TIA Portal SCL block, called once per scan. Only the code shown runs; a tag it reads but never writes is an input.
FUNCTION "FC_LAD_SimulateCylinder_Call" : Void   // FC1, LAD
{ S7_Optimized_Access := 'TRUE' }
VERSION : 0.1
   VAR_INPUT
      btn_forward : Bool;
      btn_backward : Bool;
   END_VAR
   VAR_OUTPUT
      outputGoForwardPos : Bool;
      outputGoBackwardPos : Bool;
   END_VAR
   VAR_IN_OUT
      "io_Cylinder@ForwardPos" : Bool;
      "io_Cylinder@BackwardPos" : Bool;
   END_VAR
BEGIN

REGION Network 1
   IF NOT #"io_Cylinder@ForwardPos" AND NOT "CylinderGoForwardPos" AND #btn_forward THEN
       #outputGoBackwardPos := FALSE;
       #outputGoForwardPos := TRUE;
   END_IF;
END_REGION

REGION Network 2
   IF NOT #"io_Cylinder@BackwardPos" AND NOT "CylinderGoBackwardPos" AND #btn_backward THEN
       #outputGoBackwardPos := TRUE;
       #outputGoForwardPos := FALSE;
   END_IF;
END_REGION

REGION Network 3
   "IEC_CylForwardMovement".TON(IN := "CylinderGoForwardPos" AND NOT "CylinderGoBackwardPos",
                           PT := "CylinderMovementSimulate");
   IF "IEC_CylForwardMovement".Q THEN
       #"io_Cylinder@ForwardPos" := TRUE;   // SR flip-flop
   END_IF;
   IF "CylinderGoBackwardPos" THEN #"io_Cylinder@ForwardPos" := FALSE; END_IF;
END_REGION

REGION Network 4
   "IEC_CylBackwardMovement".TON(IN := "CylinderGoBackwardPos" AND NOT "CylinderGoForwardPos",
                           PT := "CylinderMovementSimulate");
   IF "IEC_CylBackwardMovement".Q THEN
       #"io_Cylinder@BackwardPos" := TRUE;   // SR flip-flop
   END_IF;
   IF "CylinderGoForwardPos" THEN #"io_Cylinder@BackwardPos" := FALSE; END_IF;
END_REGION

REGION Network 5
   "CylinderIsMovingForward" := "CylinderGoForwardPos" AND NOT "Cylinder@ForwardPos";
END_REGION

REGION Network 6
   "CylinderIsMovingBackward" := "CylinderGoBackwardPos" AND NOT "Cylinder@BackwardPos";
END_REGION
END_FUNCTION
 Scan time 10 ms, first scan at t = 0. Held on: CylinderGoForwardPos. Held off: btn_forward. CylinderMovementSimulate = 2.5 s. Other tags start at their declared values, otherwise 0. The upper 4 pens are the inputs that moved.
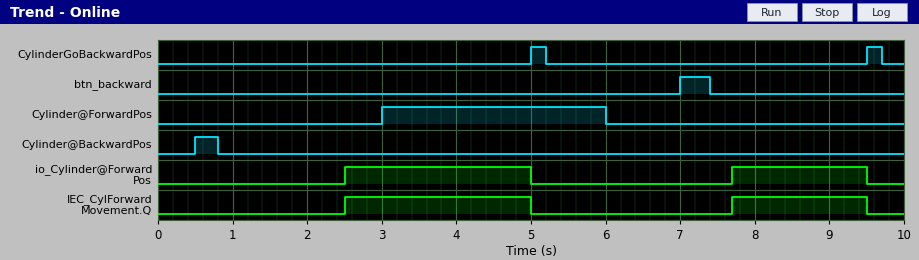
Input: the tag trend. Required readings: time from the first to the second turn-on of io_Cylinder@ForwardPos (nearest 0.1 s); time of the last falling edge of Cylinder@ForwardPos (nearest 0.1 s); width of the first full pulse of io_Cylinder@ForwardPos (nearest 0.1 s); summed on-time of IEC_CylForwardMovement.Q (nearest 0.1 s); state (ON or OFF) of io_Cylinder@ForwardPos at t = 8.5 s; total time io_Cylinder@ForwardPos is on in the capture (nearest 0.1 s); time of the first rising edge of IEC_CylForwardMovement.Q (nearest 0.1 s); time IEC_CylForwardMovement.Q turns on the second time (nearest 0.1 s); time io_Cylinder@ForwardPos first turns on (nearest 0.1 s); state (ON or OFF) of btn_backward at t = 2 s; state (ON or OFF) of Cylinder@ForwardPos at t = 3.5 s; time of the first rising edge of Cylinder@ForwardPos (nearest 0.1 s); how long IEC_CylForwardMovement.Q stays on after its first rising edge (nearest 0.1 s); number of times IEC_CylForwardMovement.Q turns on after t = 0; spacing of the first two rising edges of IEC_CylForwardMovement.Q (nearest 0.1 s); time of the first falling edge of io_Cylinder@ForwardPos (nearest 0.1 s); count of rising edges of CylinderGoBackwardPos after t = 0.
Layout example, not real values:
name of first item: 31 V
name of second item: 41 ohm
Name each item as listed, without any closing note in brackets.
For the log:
time from the first to the second turn-on of io_Cylinder@ForwardPos: 5.2 s
time of the last falling edge of Cylinder@ForwardPos: 6.0 s
width of the first full pulse of io_Cylinder@ForwardPos: 2.5 s
summed on-time of IEC_CylForwardMovement.Q: 4.3 s
state (ON or OFF) of io_Cylinder@ForwardPos at t = 8.5 s: ON
total time io_Cylinder@ForwardPos is on in the capture: 4.3 s
time of the first rising edge of IEC_CylForwardMovement.Q: 2.5 s
time IEC_CylForwardMovement.Q turns on the second time: 7.7 s
time io_Cylinder@ForwardPos first turns on: 2.5 s
state (ON or OFF) of btn_backward at t = 2 s: OFF
state (ON or OFF) of Cylinder@ForwardPos at t = 3.5 s: ON
time of the first rising edge of Cylinder@ForwardPos: 3.0 s
how long IEC_CylForwardMovement.Q stays on after its first rising edge: 2.5 s
number of times IEC_CylForwardMovement.Q turns on after t = 0: 2
spacing of the first two rising edges of IEC_CylForwardMovement.Q: 5.2 s
time of the first falling edge of io_Cylinder@ForwardPos: 5.0 s
count of rising edges of CylinderGoBackwardPos after t = 0: 2
